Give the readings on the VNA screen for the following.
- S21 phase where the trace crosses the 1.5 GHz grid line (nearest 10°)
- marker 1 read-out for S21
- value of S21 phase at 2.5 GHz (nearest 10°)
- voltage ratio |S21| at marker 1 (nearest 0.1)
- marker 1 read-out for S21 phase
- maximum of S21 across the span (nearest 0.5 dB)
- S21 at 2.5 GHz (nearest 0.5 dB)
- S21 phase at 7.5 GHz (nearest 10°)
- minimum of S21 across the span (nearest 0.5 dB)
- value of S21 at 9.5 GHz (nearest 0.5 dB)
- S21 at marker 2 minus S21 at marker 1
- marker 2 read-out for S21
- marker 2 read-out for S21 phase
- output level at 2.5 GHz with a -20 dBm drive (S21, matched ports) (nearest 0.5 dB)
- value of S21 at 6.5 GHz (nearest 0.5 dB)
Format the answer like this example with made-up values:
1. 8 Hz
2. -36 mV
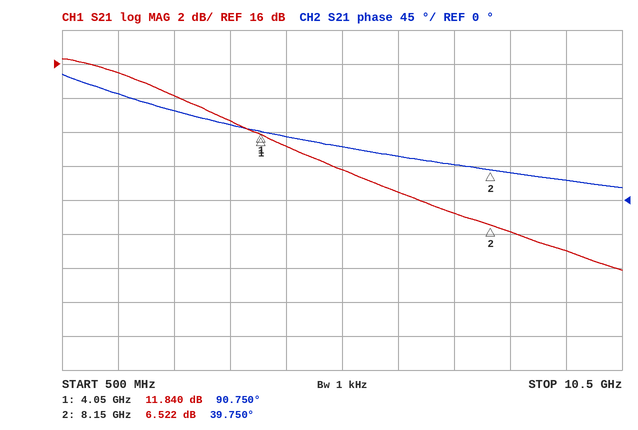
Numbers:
1. 140°
2. 11.840 dB
3. 120°
4. 3.9
5. 90.750°
6. 16.5 dB
7. 14.0 dB
8. 50°
9. 4.0 dB
10. 5.0 dB
11. -5.318 dB
12. 6.522 dB
13. 39.750°
14. -6.0 dBm
15. 8.5 dB
